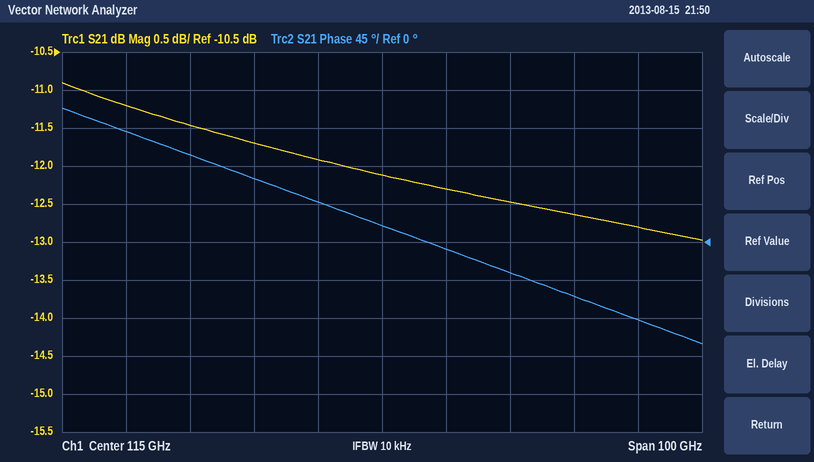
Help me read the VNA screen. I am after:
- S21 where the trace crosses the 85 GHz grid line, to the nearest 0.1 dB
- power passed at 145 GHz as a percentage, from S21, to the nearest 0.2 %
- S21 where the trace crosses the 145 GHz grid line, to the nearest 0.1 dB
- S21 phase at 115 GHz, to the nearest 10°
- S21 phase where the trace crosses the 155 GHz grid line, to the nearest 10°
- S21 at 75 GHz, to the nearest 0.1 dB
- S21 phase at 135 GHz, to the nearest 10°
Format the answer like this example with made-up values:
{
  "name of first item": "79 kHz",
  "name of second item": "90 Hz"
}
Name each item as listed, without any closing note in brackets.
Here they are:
{
  "S21 where the trace crosses the 85 GHz grid line, to the nearest 0.1 dB": "-11.5 dB",
  "power passed at 145 GHz as a percentage, from S21, to the nearest 0.2 %": "5.4 %",
  "S21 where the trace crosses the 145 GHz grid line, to the nearest 0.1 dB": "-12.6 dB",
  "S21 phase at 115 GHz, to the nearest 10°": "20°",
  "S21 phase where the trace crosses the 155 GHz grid line, to the nearest 10°": "-90°",
  "S21 at 75 GHz, to the nearest 0.1 dB": "-11.2 dB",
  "S21 phase at 135 GHz, to the nearest 10°": "-40°"
}
